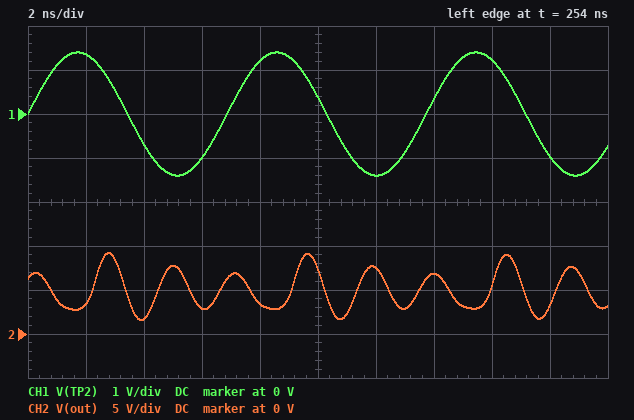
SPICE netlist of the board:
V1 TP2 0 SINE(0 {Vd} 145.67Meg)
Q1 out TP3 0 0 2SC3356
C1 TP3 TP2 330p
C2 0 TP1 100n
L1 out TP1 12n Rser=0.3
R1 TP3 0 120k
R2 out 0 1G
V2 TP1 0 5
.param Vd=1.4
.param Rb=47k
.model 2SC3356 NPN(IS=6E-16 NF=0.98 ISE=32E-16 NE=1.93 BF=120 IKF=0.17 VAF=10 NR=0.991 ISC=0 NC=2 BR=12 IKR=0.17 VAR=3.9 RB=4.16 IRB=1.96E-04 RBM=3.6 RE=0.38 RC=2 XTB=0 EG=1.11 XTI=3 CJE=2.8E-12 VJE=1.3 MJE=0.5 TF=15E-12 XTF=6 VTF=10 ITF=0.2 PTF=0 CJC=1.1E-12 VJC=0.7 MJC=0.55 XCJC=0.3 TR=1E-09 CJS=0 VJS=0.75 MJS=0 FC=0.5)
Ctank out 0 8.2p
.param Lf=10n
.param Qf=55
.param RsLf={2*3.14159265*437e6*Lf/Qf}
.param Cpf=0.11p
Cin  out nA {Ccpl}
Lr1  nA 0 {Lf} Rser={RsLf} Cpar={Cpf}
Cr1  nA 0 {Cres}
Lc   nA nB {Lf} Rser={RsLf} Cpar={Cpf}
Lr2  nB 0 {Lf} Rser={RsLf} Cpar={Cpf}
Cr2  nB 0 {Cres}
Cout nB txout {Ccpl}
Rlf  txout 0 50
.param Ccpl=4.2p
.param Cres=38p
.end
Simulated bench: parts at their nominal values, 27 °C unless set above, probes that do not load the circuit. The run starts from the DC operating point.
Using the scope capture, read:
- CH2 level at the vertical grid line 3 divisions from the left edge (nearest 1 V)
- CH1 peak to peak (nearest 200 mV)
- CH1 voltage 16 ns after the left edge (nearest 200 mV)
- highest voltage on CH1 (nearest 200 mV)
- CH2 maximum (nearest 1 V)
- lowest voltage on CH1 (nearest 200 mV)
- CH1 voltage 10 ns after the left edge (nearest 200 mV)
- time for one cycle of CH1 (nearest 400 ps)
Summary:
3 V
2.8 V
1.2 V
1.4 V
9 V
-1.4 V
400 mV
6.8 ns
